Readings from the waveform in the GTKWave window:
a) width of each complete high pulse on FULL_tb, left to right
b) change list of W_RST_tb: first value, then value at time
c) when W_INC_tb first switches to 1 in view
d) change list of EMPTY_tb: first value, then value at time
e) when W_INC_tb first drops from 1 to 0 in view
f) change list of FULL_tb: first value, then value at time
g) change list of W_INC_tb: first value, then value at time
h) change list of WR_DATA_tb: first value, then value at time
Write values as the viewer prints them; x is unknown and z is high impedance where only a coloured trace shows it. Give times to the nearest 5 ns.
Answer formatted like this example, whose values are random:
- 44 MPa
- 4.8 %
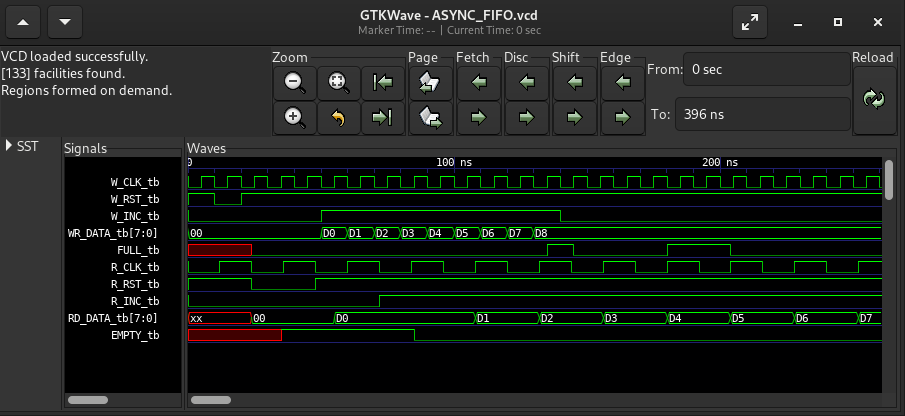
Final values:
- 10 ns, 25 ns
- 1, 0 at 10 ns, 1 at 20 ns
- 50 ns
- x, 1 at 35 ns, 0 at 85 ns
- 140 ns
- x, 0 at 25 ns, 1 at 135 ns, 0 at 145 ns, 1 at 180 ns, 0 at 205 ns
- 0, 1 at 50 ns, 0 at 140 ns
- 00, D0 at 50 ns, D1 at 60 ns, D2 at 70 ns, D3 at 80 ns, D4 at 90 ns, D5 at 100 ns, D6 at 110 ns, D7 at 120 ns, D8 at 130 ns
